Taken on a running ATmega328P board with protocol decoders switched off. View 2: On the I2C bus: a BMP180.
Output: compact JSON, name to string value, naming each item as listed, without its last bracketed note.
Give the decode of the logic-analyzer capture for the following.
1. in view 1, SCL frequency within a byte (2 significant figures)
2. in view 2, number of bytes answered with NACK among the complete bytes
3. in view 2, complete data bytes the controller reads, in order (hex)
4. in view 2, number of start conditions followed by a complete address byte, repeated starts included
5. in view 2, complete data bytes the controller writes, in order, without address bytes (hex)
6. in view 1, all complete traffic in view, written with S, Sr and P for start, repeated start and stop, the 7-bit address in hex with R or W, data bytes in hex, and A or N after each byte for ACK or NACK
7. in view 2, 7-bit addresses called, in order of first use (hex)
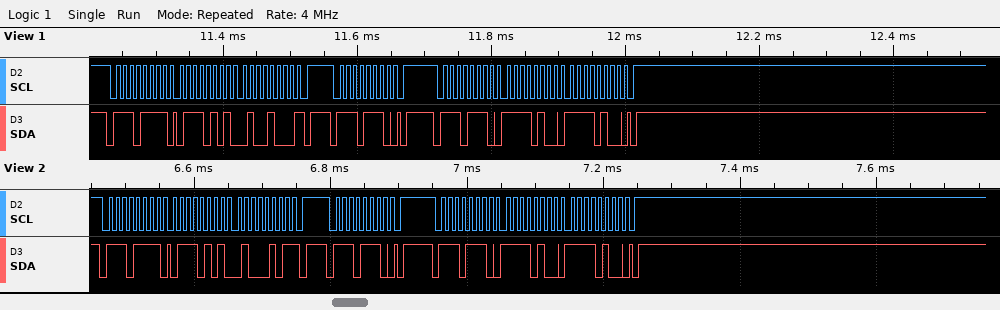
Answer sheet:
{"in view 1, SCL frequency within a byte": "100 kHz", "in view 2, number of bytes answered with NACK among the complete bytes": "1", "in view 2, complete data bytes the controller reads, in order": "75 45", "in view 2, number of start conditions followed by a complete address byte, repeated starts included": "3", "in view 2, complete data bytes the controller writes, in order, without address bytes": "F4 F4", "in view 1, all complete traffic in view, written with S, Sr and P for start, repeated start and stop, the 7-bit address in hex with R or W, data bytes in hex, and A or N after each byte for ACK or NACK": "S 77R A 75 A 48 N P S 77W A P S 77W A F4 A F4 A P", "in view 2, 7-bit addresses called, in order of first use": "0x77"}
